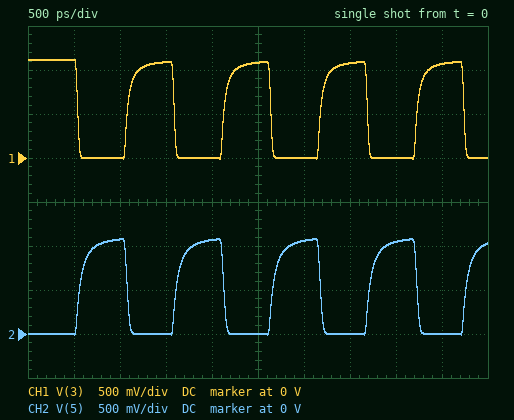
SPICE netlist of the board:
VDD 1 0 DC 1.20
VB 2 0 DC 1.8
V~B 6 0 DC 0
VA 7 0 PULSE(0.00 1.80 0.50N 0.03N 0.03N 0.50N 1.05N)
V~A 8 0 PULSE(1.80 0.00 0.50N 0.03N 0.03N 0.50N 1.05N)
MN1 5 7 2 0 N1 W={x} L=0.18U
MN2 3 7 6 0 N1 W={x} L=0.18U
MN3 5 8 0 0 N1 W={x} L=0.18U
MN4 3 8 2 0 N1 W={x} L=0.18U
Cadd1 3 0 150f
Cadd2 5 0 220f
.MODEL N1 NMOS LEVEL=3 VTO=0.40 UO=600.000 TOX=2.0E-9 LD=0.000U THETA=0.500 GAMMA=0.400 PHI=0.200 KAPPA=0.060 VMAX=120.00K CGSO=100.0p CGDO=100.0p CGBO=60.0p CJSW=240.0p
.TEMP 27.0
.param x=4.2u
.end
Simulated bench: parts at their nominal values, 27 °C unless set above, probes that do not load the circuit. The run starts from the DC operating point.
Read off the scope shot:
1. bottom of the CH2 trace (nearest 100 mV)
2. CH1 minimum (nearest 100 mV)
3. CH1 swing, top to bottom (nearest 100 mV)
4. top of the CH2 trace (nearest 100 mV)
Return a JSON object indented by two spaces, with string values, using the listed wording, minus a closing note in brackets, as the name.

{
  "bottom of the CH2 trace": "0 V",
  "CH1 minimum": "0 V",
  "CH1 swing, top to bottom": "1.1 V",
  "top of the CH2 trace": "1.1 V"
}
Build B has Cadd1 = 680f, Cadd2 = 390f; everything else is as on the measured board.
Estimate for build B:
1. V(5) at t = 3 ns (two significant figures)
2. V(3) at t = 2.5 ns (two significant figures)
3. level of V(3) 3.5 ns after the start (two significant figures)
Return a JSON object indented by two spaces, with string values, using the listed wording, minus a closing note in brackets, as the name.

{
  "V(5) at t = 3 ns": "1.0 V",
  "V(3) at t = 2.5 ns": "900 mV",
  "level of V(3) 3.5 ns after the start": "860 mV"
}
